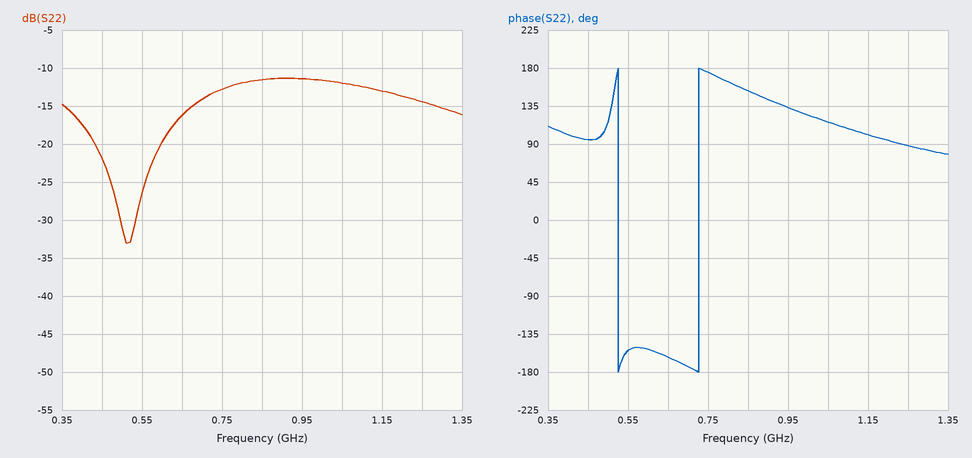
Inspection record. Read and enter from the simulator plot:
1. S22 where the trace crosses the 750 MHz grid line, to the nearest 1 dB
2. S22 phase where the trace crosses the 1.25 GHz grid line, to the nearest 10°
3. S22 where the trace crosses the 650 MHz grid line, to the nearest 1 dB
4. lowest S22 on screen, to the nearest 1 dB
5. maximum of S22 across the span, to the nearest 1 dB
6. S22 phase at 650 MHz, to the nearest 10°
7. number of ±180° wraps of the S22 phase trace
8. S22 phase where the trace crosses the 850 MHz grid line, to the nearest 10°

-13 dB
90°
-16 dB
-33 dB
-11 dB
-160°
2
150°
